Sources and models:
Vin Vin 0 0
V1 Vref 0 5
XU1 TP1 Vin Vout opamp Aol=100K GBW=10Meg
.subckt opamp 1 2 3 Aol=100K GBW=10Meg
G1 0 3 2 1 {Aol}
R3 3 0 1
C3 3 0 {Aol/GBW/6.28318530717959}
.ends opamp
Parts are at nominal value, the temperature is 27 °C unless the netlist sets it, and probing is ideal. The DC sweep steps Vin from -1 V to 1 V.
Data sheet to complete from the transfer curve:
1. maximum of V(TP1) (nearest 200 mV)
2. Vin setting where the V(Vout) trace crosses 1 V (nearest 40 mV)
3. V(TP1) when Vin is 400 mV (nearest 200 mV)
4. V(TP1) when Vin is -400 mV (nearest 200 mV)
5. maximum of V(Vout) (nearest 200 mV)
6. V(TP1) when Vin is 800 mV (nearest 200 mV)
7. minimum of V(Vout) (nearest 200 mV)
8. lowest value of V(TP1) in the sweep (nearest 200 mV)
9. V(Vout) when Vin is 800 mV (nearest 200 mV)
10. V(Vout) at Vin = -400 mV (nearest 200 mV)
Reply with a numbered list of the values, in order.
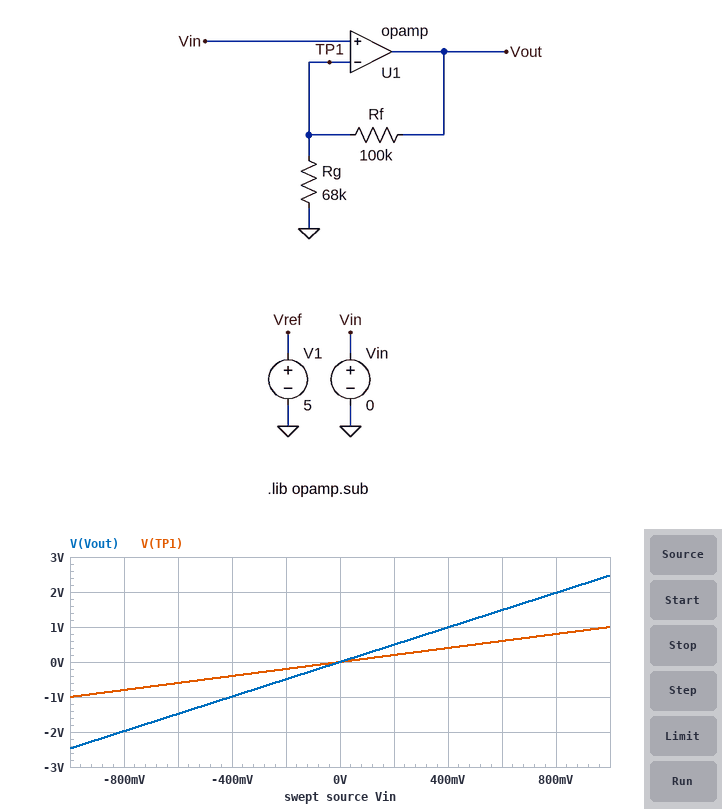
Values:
1. 1.0 V
2. 400 mV
3. 400 mV
4. -400 mV
5. 2.4 V
6. 800 mV
7. -2.4 V
8. -1.0 V
9. 2.0 V
10. -1.0 V
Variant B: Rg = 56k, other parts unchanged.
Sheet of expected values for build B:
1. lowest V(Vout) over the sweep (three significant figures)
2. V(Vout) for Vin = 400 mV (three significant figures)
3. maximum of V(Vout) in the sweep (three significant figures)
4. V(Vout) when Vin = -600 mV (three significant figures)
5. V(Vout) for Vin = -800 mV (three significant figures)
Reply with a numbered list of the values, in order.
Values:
1. -2.79 V
2. 1.11 V
3. 2.79 V
4. -1.67 V
5. -2.23 V
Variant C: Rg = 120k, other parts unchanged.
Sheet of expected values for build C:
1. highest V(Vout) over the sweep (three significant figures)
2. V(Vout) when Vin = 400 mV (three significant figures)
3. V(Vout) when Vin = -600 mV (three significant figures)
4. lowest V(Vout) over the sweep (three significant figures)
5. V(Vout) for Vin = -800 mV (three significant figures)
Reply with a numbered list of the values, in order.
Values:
1. 1.83 V
2. 733 mV
3. -1.10 V
4. -1.83 V
5. -1.47 V
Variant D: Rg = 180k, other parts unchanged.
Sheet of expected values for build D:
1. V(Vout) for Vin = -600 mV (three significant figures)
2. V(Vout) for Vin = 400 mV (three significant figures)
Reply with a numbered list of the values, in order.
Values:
1. -933 mV
2. 622 mV
